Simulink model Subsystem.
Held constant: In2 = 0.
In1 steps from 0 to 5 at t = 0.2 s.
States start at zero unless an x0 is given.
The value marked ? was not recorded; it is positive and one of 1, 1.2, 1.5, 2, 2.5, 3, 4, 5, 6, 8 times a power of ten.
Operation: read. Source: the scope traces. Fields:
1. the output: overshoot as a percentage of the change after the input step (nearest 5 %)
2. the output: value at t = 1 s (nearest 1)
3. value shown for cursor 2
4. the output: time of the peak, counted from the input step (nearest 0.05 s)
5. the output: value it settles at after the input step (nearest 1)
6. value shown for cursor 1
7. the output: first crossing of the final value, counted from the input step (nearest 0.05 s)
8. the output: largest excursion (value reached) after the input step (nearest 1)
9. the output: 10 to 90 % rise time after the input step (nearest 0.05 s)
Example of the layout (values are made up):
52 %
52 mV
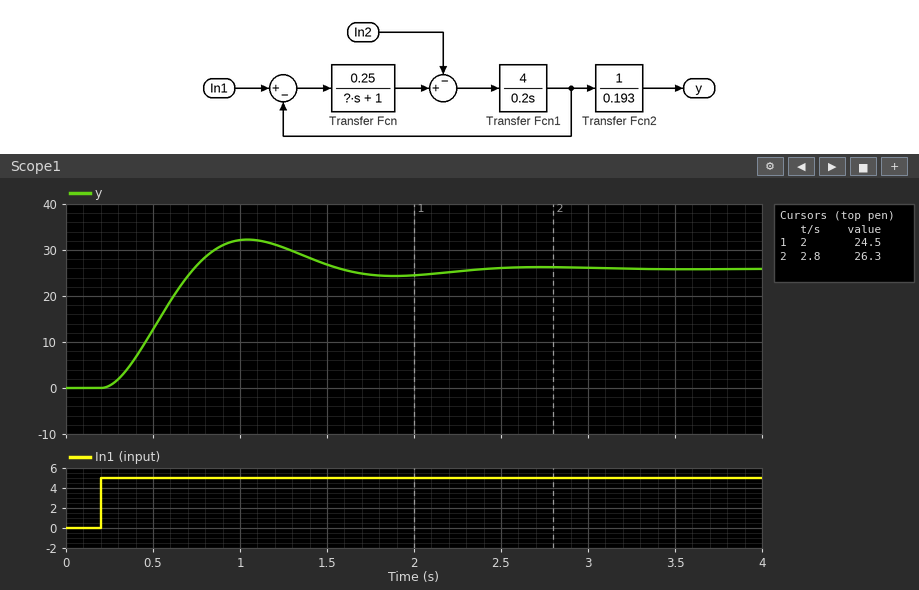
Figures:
25 %
32
26.3
0.85 s
26
24.5
0.55 s
32
0.35 s
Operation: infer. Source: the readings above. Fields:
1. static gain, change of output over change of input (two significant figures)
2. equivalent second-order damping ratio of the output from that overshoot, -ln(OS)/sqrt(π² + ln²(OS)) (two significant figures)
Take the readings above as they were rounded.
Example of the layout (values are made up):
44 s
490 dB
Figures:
5.2
0.40
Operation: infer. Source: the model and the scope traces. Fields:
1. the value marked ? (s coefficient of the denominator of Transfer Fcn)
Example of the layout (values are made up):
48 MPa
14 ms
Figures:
0.3
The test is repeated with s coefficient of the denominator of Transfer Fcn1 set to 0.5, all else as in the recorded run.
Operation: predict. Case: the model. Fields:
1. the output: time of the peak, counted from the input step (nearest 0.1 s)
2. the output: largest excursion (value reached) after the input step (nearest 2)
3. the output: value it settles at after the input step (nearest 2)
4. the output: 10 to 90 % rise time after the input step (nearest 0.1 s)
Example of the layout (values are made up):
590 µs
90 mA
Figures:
1.6 s
28
26
0.8 s
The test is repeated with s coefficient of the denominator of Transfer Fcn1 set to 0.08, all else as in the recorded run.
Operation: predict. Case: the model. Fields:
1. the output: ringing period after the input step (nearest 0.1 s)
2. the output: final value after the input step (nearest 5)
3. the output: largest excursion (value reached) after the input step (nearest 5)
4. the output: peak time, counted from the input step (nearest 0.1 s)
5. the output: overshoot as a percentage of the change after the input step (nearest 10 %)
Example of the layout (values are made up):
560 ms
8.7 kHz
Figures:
1.0 s
25
35
0.5 s
40 %
